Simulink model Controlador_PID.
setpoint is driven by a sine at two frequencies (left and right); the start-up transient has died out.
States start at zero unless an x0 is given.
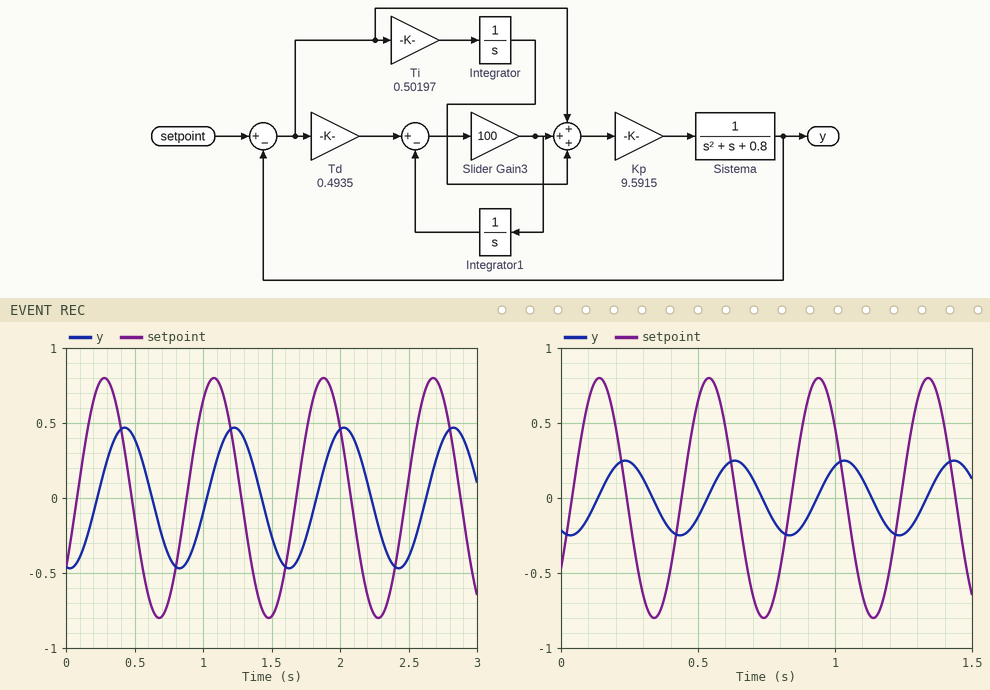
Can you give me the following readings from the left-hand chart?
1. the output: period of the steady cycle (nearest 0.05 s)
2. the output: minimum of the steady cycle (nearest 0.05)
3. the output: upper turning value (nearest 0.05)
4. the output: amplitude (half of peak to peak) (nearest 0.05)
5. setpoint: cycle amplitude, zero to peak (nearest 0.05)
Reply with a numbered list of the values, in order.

1. 0.80 s
2. -0.45
3. 0.45
4. 0.45
5. 0.80
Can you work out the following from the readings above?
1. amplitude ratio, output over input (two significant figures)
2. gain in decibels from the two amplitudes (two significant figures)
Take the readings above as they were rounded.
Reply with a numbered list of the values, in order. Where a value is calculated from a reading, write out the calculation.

1. 0.45 / 0.8 = 0.56
2. 20 log10(0.45 / 0.8) = -5.0 dB
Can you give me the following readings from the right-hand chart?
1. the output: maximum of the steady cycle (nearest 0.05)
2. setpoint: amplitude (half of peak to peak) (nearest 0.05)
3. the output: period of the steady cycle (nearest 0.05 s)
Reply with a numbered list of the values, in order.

1. 0.25
2. 0.80
3. 0.40 s
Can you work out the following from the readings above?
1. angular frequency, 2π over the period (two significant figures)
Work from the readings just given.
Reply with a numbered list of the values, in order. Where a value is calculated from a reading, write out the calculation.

1. 2π / 0.4 = 16 rad/s
